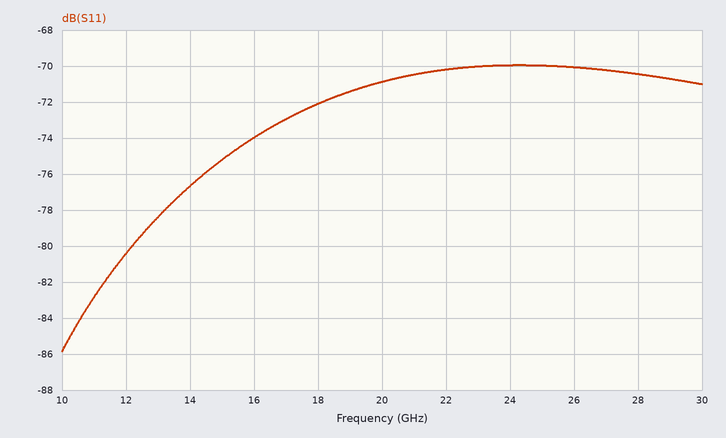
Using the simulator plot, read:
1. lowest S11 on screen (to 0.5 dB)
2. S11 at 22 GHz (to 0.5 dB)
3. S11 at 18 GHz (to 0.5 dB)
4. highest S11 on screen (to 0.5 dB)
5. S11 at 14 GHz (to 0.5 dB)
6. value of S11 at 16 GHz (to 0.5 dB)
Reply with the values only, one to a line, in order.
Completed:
-86.0 dB
-70.0 dB
-72.0 dB
-70.0 dB
-76.5 dB
-74.0 dB
